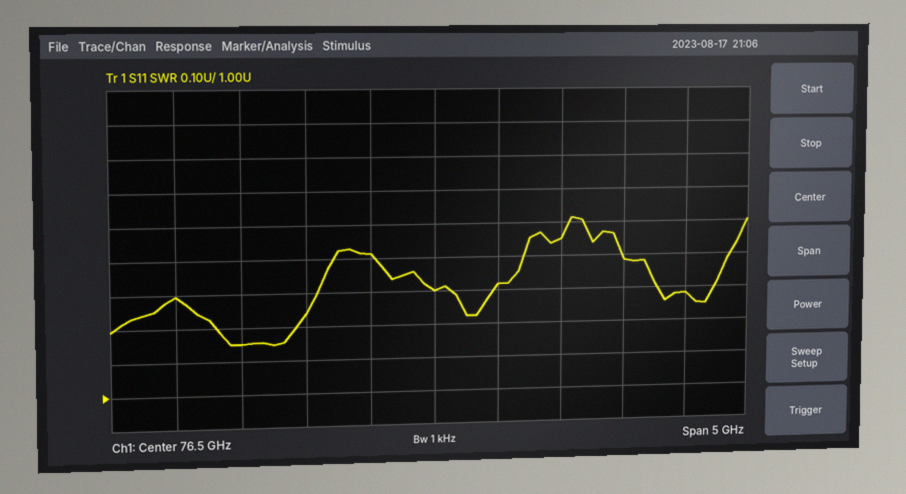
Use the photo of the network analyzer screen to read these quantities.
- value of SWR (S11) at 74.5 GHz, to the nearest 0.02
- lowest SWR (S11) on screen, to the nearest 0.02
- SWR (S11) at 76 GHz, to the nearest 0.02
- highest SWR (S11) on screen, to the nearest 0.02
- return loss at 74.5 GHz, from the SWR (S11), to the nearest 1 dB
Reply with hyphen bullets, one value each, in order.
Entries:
- 1.30
- 1.14
- 1.42
- 1.52
- 18 dB
